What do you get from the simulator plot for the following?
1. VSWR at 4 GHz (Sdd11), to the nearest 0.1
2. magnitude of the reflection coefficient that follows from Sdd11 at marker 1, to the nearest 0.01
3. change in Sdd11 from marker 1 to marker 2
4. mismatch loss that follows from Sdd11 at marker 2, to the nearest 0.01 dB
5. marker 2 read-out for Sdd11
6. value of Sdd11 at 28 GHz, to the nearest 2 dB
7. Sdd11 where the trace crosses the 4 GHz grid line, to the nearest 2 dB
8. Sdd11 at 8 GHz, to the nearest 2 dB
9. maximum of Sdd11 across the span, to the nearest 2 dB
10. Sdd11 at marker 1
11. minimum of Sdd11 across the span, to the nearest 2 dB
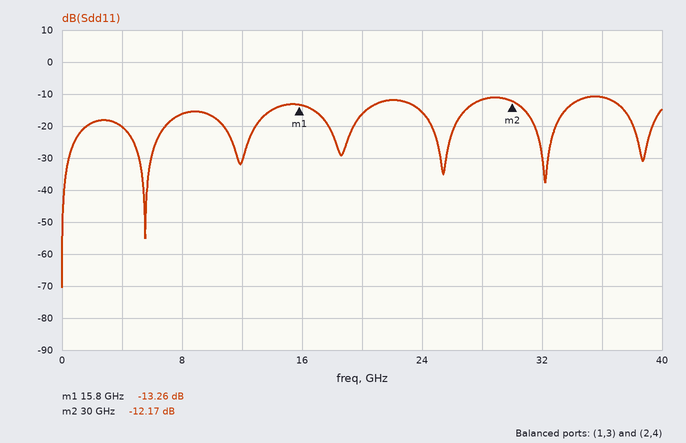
1.2
0.22
1.09 dB
0.27 dB
-12.17 dB
-12 dB
-20 dB
-16 dB
-10 dB
-13.26 dB
-70 dB
